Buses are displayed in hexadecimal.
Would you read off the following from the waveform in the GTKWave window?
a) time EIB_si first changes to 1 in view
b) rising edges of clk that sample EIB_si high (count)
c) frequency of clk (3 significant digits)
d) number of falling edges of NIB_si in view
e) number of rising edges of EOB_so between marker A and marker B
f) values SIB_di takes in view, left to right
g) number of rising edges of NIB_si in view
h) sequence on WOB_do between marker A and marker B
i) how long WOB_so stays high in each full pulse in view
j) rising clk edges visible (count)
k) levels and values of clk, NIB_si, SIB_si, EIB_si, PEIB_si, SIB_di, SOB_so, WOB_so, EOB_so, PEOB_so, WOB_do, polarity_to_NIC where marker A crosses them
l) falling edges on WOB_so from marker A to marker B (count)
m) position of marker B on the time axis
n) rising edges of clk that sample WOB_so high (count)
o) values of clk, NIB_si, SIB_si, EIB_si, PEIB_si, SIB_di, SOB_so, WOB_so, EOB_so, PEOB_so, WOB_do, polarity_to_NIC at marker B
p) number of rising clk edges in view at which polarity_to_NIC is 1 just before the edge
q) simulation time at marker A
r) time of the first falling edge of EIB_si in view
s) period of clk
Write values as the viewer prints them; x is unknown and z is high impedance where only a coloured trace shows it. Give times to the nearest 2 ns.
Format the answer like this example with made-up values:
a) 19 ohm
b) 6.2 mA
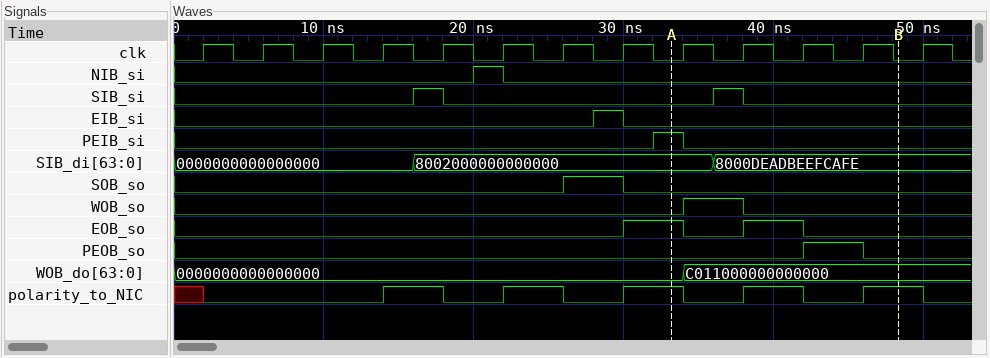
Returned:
a) 28 ns
b) 1
c) 250 MHz
d) 1
e) 1
f) 0000000000000000, 8002000000000000, 8000DEADBEEFCAFE
g) 1
h) 0000000000000000, C011000000000000
i) 4 ns
j) 13
k) clk=0, NIB_si=0, SIB_si=0, EIB_si=0, PEIB_si=1, SIB_di=8002000000000000, SOB_so=0, WOB_so=0, EOB_so=1, PEOB_so=0, WOB_do=0000000000000000, polarity_to_NIC=1
l) 1
m) 48 ns
n) 1
o) clk=0, NIB_si=0, SIB_si=0, EIB_si=0, PEIB_si=0, SIB_di=8000DEADBEEFCAFE, SOB_so=0, WOB_so=0, EOB_so=0, PEOB_so=0, WOB_do=C011000000000000, polarity_to_NIC=1
p) 5
q) 34 ns
r) 30 ns
s) 4 ns
